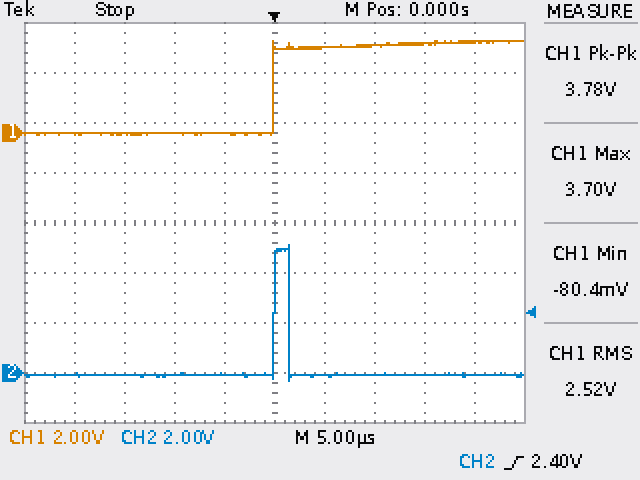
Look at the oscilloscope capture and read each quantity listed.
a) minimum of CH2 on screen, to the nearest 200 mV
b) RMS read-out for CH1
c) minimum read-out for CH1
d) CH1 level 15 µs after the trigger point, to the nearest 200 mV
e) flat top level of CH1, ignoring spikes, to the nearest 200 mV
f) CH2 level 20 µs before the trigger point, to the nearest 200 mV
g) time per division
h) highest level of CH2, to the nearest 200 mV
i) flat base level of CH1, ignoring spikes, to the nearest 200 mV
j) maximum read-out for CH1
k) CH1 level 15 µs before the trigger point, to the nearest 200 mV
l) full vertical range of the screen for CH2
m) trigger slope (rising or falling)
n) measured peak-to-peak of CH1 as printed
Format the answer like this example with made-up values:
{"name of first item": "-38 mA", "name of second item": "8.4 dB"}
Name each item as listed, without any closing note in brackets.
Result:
{"minimum of CH2 on screen, to the nearest 200 mV": "-400 mV", "RMS read-out for CH1": "2.52 V", "minimum read-out for CH1": "-80.4 mV", "CH1 level 15 µs after the trigger point, to the nearest 200 mV": "3.6 V", "flat top level of CH1, ignoring spikes, to the nearest 200 mV": "3.6 V", "CH2 level 20 µs before the trigger point, to the nearest 200 mV": "0.0 V", "time per division": "5 µs", "highest level of CH2, to the nearest 200 mV": "5.2 V", "flat base level of CH1, ignoring spikes, to the nearest 200 mV": "0.0 V", "maximum read-out for CH1": "3.70 V", "CH1 level 15 µs before the trigger point, to the nearest 200 mV": "0.0 V", "full vertical range of the screen for CH2": "16 V", "trigger slope": "rising", "measured peak-to-peak of CH1 as printed": "3.78 V"}
